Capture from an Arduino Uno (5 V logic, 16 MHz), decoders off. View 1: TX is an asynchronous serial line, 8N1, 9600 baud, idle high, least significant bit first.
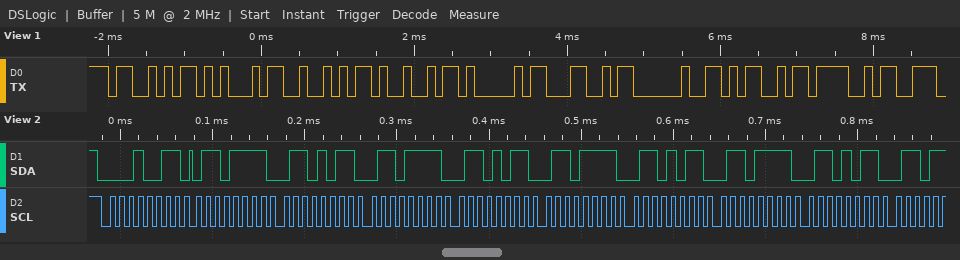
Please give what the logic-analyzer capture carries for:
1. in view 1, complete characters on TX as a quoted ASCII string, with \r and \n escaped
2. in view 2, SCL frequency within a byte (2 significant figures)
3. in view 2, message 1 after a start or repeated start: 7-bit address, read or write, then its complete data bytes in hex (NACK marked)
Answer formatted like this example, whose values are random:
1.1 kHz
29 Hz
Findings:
"SERIAL MO"
100 kHz
0x09 read: 6F 6B 6F 6B 6F 6B 6F 6B
